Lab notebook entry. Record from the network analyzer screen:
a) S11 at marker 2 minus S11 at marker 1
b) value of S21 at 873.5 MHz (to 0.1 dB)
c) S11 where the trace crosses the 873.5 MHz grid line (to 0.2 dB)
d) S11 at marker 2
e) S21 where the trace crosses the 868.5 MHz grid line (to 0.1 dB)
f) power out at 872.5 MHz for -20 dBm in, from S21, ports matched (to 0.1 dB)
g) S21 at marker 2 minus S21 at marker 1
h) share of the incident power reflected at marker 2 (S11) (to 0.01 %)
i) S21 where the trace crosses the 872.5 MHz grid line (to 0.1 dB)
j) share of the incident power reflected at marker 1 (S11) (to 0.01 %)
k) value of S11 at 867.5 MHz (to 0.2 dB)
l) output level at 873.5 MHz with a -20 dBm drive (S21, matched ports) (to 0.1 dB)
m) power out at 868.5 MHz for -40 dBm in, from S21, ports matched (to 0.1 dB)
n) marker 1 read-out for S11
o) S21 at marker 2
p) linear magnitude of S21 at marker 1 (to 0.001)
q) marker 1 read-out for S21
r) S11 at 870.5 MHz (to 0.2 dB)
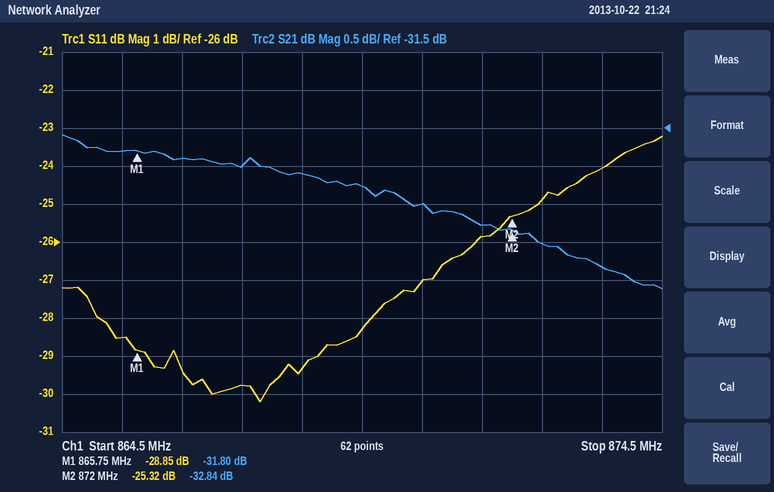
3.53 dB
-33.3 dB
-24.0 dB
-25.32 dB
-32.1 dB
-53.0 dBm
-1.04 dB
0.29 %
-33.0 dB
0.13 %
-29.8 dB
-53.3 dBm
-72.1 dBm
-28.85 dB
-32.84 dB
0.026
-31.80 dB
-27.0 dB
